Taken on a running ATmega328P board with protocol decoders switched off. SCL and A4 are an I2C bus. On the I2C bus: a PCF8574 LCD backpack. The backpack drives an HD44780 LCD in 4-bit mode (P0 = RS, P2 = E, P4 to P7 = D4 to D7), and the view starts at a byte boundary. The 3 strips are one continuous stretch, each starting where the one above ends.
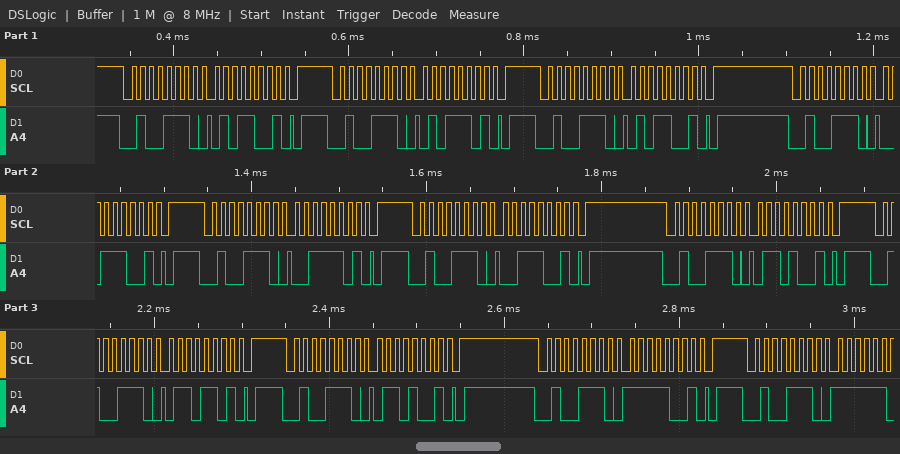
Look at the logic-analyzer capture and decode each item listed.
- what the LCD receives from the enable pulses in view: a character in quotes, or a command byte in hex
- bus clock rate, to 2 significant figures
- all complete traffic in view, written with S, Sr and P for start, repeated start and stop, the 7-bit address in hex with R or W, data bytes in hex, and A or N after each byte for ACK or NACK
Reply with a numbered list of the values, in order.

1. 'S'
2. 100 kHz
3. S 27W A 59 A P S 27W A 5D A P S 27W A 59 A P S 27W A 39 A P S 27W A 3D A P S 27W A 39 A P S 27W A 69 A P S 27W A 6D A P S 27W A 69 A P S 27W A F9 A P S 27W A
